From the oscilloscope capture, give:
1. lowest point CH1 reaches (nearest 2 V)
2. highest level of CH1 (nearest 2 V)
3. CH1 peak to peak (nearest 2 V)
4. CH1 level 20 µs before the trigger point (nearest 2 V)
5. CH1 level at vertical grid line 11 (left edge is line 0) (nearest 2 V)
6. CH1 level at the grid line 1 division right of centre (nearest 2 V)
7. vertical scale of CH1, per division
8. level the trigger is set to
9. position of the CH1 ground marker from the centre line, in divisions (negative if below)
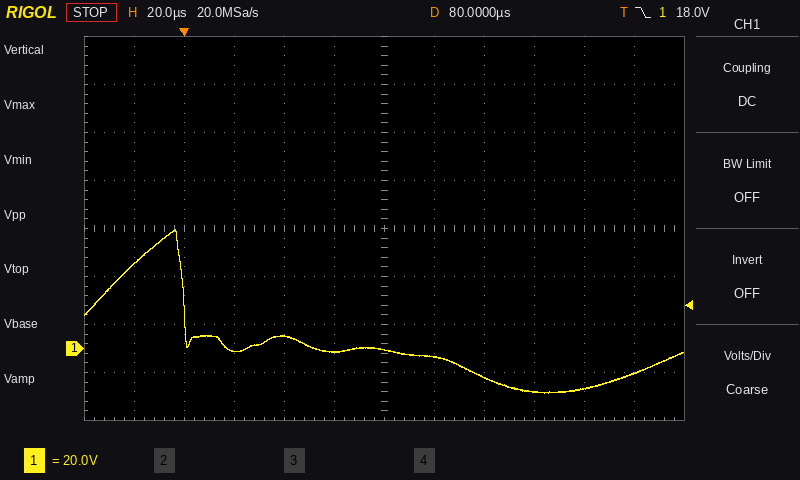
-18 V
50 V
68 V
36 V
-10 V
-4 V
20 V
18.0 V
-2.5 div
